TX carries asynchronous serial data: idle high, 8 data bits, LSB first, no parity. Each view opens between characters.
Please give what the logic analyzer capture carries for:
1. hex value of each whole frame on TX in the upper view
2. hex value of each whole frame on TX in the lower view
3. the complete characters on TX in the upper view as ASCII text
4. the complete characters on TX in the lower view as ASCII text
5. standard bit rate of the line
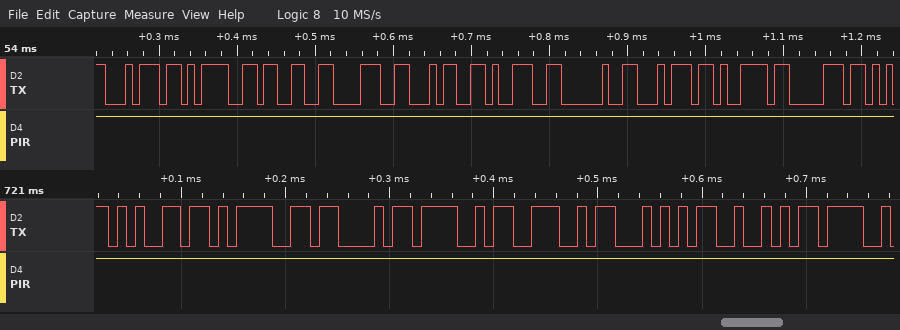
74, 3D, 33, 38, 34, 39, 20, 74, 79, 70
65, 3D, 43, 4F, 4E, 54, 52
"t=3849 typ"
"e=CONTR"
115200 baud
